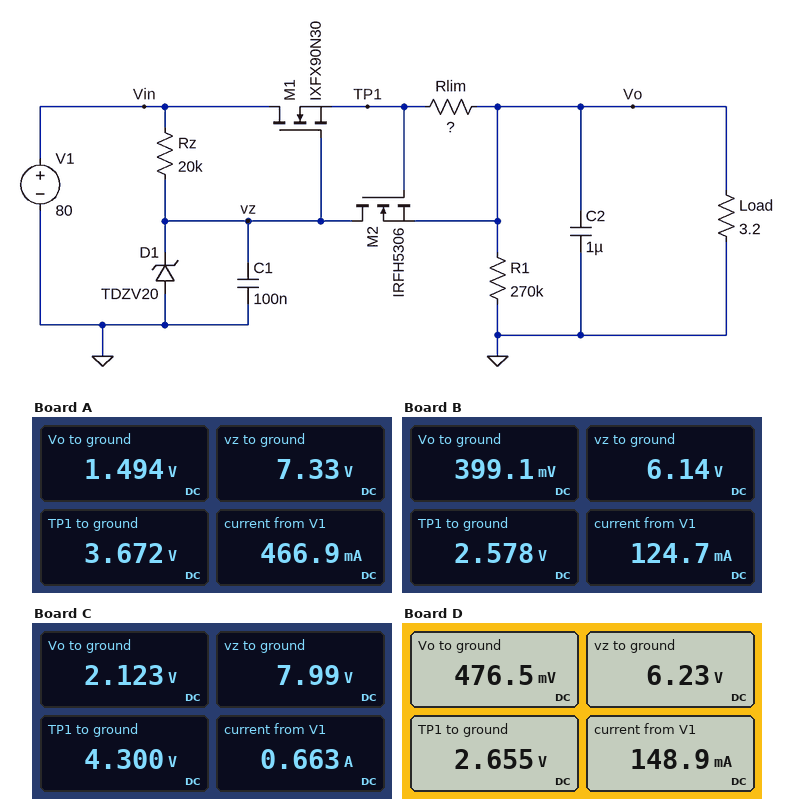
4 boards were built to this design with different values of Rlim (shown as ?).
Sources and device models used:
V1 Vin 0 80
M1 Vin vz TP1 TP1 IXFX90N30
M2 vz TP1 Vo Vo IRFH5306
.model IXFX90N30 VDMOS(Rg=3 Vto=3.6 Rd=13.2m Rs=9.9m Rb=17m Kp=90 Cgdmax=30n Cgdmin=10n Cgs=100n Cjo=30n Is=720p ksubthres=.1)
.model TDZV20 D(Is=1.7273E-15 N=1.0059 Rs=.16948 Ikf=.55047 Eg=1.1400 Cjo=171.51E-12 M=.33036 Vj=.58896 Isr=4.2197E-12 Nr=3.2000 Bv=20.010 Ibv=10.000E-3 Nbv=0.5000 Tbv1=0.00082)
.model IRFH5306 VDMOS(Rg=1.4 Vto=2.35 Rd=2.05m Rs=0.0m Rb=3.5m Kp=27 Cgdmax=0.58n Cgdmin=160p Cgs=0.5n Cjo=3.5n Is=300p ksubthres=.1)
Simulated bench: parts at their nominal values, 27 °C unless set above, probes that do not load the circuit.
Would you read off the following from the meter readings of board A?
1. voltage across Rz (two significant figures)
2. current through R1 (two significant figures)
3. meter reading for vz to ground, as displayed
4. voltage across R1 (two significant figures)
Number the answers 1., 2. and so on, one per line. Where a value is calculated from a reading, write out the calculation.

1. 80 V - 7.33 V = 73 V
2. (1.494 V) / 270 kΩ = 5.5 µA
3. 7.33 V
4. 1.494 V = 1.5 V
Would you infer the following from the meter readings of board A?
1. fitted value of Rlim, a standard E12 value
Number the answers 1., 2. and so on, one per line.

1. 4.7 Ω
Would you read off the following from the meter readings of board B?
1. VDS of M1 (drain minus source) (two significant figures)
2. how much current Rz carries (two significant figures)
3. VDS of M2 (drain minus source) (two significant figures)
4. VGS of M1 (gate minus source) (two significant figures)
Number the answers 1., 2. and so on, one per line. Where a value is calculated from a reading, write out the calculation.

1. 80 V - 2.578 V = 77 V
2. (80 V - 6.14 V) / 20 kΩ = 3.7 mA
3. 6.14 V - 399.1 mV = 5.7 V
4. 6.14 V - 2.578 V = 3.6 V
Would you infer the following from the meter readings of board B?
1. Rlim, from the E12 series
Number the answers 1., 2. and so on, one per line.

1. 18 Ω
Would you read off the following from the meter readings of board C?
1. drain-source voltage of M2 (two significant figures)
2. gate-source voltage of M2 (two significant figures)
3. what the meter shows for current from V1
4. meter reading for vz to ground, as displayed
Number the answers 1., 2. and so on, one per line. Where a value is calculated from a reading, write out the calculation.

1. 7.99 V - 2.123 V = 5.9 V
2. 4.3 V - 2.123 V = 2.2 V
3. 0.663 A
4. 7.99 V
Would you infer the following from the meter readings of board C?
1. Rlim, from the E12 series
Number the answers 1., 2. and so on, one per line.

1. 3.3 Ω
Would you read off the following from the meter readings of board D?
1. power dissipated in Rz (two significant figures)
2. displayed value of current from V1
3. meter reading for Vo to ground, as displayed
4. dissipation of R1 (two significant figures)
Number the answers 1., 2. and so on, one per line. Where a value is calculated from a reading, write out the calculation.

1. (80 V - 6.23 V)^2 / 20 kΩ = 270 mW
2. 148.9 mA
3. 476.5 mV
4. (476.5 mV)^2 / 270 kΩ = 840 nW
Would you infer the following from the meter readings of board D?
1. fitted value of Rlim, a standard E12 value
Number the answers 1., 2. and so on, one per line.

1. 15 Ω
